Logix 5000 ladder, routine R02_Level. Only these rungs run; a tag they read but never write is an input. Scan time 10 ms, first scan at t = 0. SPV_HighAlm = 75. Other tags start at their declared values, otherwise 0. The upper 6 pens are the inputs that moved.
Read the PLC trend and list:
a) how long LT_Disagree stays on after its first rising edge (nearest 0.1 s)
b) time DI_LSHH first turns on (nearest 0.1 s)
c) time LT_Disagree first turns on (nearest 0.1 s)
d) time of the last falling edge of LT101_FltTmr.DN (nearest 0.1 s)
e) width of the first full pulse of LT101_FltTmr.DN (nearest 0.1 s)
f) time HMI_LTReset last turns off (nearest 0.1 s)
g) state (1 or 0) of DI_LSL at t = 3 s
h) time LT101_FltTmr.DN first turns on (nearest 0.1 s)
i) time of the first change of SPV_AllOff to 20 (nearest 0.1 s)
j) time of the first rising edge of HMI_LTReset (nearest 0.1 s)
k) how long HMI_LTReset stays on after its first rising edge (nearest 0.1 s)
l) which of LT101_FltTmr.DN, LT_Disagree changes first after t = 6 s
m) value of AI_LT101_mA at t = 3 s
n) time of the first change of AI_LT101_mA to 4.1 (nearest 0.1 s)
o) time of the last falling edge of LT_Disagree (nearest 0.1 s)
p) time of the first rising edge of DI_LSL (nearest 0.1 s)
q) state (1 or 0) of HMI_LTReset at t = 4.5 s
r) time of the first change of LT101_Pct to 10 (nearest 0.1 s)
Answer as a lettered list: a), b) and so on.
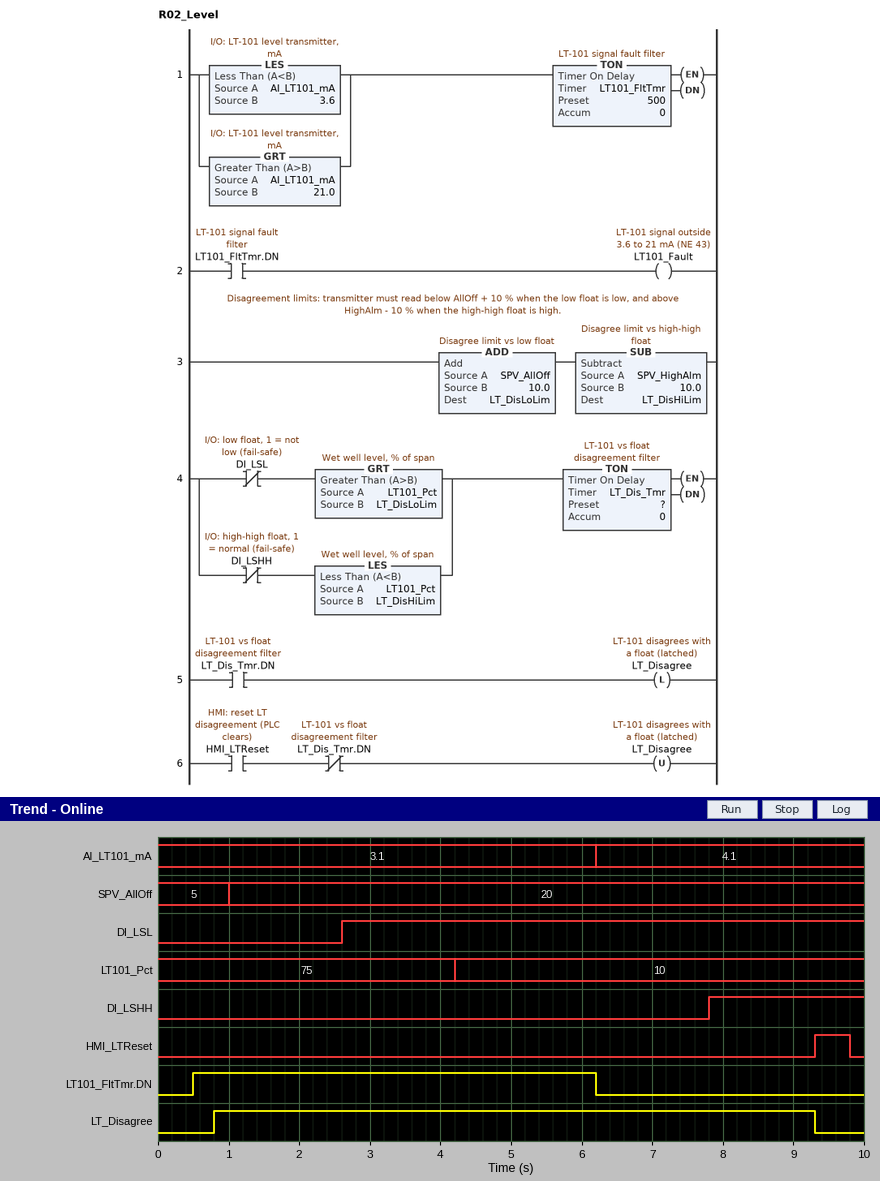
a) 8.5 s
b) 7.8 s
c) 0.8 s
d) 6.2 s
e) 5.7 s
f) 9.8 s
g) 1
h) 0.5 s
i) 1.0 s
j) 9.3 s
k) 0.5 s
l) LT101_FltTmr.DN
m) 3.1
n) 6.2 s
o) 9.3 s
p) 2.6 s
q) 0
r) 4.2 s
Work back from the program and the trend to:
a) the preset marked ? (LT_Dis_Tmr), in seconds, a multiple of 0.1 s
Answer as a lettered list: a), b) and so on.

a) 0.8 s
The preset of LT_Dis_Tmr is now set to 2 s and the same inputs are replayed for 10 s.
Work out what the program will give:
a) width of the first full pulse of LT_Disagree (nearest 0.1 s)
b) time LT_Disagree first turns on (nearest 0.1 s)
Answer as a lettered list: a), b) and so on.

a) 7.3 s
b) 2.0 s
